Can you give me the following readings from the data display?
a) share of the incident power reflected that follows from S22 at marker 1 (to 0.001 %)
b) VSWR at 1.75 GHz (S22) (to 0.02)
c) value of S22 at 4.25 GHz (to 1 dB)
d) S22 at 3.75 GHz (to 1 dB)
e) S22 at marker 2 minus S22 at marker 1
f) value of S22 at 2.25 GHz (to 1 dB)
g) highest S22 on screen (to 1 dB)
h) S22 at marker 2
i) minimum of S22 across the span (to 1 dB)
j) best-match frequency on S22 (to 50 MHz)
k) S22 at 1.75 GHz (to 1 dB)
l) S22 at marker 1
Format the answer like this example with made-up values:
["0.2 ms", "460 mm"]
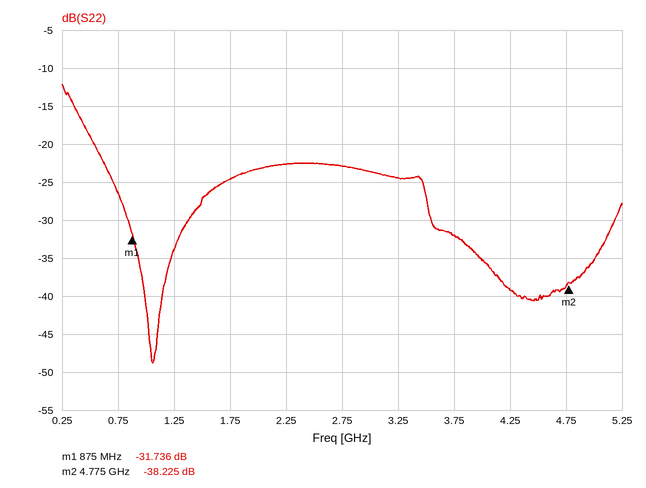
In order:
["0.067 %", "1.12", "-39 dB", "-32 dB", "-6.489 dB", "-23 dB", "-12 dB", "-38.225 dB", "-49 dB", "1.05 GHz", "-25 dB", "-31.736 dB"]
